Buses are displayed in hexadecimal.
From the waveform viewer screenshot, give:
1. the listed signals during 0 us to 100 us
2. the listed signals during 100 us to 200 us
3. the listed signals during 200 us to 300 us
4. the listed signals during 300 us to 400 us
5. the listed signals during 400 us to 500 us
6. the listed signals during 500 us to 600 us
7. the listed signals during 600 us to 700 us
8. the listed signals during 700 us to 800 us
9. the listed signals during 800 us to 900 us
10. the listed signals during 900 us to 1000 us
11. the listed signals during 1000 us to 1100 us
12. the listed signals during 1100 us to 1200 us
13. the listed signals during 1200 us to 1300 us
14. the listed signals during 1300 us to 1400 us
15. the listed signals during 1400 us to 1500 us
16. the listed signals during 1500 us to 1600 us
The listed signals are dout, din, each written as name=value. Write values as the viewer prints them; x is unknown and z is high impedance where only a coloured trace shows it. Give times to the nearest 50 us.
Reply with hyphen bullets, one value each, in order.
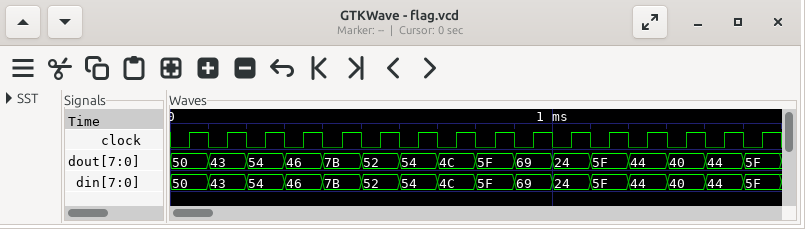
- dout=50, din=50
- dout=43, din=43
- dout=54, din=54
- dout=46, din=46
- dout=7B, din=7B
- dout=52, din=52
- dout=54, din=54
- dout=4C, din=4C
- dout=5F, din=5F
- dout=69, din=69
- dout=24, din=24
- dout=5F, din=5F
- dout=44, din=44
- dout=40, din=40
- dout=44, din=44
- dout=5F, din=5F
